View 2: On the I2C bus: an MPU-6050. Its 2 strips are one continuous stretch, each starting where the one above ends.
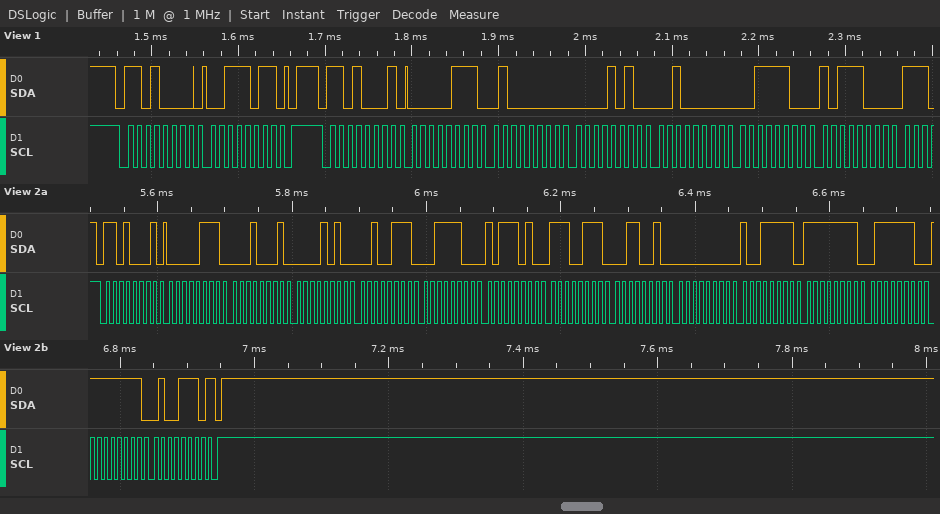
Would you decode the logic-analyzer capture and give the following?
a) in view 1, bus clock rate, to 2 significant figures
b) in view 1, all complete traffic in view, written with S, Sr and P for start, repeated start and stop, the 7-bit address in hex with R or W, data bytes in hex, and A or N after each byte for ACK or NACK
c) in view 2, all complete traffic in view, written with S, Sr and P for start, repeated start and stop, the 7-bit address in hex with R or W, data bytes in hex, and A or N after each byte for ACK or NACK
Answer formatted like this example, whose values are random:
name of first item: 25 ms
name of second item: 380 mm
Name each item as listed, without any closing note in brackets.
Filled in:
in view 1, bus clock rate, to 2 significant figures: 100 kHz
in view 1, all complete traffic in view, written with S, Sr and P for start, repeated start and stop, the 7-bit address in hex with R or W, data bytes in hex, and A or N after each byte for ACK or NACK: S 68W A 3B A P S 68R A 07 A 40 A 0A A 20 A 3C A B8 A
in view 2, all complete traffic in view, written with S, Sr and P for start, repeated start and stop, the 7-bit address in hex with R or W, data bytes in hex, and A or N after each byte for ACK or NACK: S 68R A 07 A 11 A 0A A 27 A 3C A BA A E7 A 32 A 00 A 9F A FF A 7E A FF A 4E N P
